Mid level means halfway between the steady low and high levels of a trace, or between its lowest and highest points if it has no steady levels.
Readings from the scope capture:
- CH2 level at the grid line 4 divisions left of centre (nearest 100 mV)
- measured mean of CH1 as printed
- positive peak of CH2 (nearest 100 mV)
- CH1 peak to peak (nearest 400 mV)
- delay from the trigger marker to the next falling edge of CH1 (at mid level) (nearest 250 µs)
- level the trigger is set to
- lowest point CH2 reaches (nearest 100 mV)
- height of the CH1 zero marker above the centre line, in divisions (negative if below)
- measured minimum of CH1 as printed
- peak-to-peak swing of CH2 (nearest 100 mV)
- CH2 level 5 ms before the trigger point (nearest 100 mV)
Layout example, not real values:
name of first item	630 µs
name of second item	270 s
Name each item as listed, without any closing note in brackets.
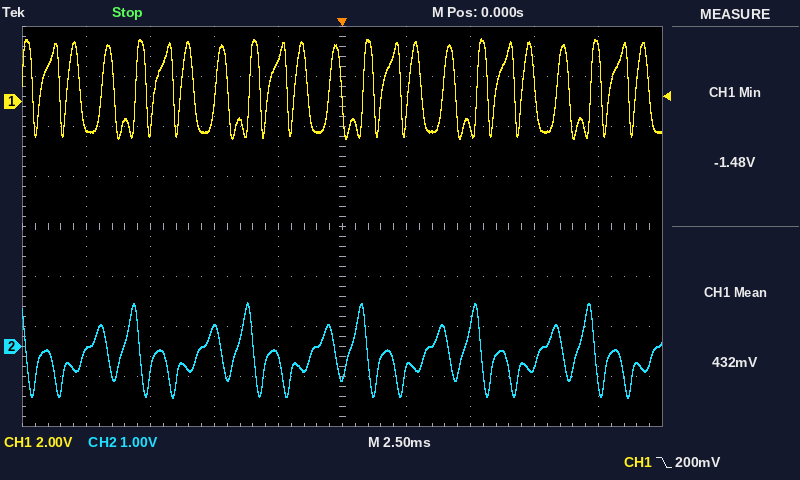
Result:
CH2 level at the grid line 4 divisions left of centre	-100 mV
measured mean of CH1 as printed	432 mV
positive peak of CH2	900 mV
CH1 peak to peak	4.0 V
delay from the trigger marker to the next falling edge of CH1 (at mid level)	1.25 ms
level the trigger is set to	200 mV
lowest point CH2 reaches	-1.0 V
height of the CH1 zero marker above the centre line, in divisions	+2.5 div
measured minimum of CH1 as printed	-1.48 V
peak-to-peak swing of CH2	1.9 V
CH2 level 5 ms before the trigger point	400 mV
